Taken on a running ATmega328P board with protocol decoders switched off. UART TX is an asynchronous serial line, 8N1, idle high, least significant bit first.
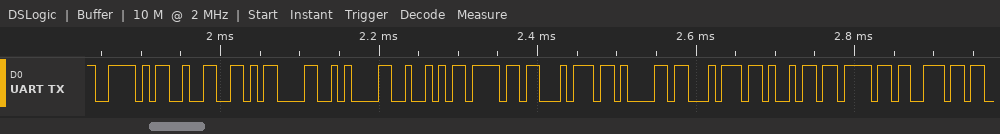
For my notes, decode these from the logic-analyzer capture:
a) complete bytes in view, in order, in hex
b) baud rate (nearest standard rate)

0x5E 0x32 0x0D 0x0A 0x52 0x6F 0x74 0x61 0x74 0x69 0x6F 0x6E
115200 baud
